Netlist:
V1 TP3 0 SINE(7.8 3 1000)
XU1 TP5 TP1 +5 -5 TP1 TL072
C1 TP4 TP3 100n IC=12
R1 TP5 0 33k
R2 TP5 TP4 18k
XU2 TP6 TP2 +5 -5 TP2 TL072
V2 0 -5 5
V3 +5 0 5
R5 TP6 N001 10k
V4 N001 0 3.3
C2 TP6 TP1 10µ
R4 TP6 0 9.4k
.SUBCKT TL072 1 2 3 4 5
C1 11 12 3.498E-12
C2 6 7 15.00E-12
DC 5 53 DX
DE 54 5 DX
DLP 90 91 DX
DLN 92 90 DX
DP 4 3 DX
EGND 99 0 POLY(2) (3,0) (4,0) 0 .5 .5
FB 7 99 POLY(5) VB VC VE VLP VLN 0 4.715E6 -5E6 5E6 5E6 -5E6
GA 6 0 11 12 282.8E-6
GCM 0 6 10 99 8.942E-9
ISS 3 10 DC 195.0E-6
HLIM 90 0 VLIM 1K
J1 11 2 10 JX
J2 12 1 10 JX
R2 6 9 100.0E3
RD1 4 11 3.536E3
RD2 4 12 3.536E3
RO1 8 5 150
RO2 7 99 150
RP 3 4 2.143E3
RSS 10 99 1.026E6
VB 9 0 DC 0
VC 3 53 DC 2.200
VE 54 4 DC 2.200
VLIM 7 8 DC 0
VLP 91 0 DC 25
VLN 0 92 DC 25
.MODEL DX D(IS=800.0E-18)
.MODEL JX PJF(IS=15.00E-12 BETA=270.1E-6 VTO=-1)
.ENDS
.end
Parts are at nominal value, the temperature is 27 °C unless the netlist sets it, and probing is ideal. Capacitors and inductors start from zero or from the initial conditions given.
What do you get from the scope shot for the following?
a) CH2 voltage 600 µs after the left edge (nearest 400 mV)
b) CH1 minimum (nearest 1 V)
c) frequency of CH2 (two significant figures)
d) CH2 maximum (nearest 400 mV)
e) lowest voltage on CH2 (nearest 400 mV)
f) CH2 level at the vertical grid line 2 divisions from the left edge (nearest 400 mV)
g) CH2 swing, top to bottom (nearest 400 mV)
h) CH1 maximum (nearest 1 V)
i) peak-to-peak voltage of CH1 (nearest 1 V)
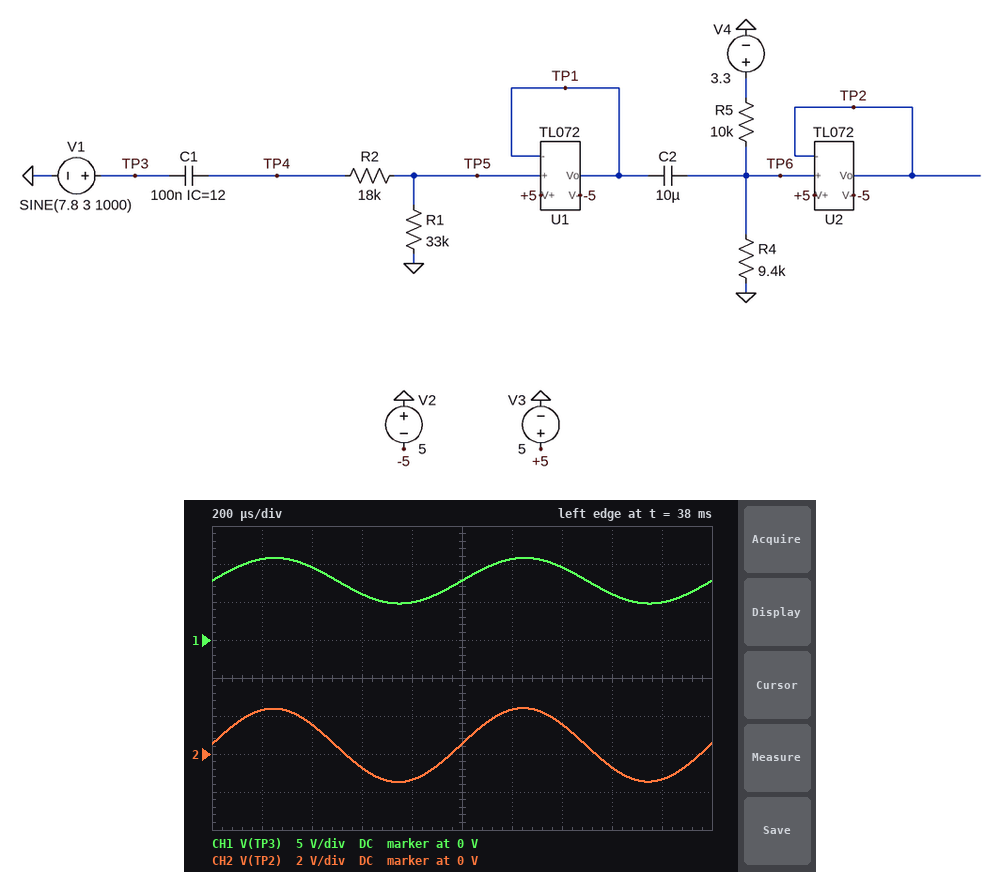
-800 mV
5 V
1.0 kHz
2.4 V
-1.6 V
1.6 V
4.0 V
11 V
6 V
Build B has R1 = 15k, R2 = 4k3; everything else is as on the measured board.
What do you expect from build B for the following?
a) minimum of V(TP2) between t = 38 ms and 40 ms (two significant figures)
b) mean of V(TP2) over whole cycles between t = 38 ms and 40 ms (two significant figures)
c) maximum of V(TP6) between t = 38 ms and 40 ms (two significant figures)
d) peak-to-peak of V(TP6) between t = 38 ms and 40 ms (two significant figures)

-1.6 V
730 mV
3.1 V
4.7 V
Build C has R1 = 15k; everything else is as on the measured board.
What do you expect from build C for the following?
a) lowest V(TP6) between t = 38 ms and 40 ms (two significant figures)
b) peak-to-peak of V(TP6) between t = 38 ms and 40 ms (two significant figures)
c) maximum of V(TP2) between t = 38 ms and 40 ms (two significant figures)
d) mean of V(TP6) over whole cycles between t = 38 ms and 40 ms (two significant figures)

-700 mV
2.7 V
2.0 V
660 mV
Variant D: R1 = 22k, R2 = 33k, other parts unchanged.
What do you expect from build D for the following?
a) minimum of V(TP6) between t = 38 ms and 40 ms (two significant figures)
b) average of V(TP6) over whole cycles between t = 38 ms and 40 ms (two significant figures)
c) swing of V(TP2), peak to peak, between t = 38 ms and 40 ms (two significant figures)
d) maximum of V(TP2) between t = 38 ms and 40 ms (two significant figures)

-680 mV
530 mV
2.4 V
1.7 V
